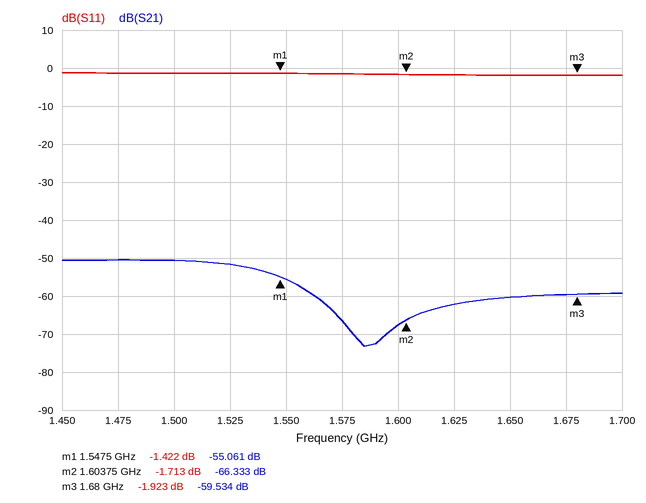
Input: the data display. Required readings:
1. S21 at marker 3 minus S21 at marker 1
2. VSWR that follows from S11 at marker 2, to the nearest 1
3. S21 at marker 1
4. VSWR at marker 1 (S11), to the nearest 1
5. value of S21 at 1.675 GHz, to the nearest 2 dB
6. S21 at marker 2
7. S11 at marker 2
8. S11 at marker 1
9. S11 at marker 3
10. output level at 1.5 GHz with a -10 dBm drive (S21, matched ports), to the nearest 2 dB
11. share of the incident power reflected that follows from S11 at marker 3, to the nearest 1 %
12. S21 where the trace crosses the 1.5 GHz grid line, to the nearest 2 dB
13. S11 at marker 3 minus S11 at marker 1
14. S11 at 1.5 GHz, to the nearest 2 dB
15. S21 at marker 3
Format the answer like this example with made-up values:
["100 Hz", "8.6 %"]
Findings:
["-4.473 dB", "10", "-55.061 dB", "12", "-60 dB", "-66.333 dB", "-1.713 dB", "-1.422 dB", "-1.923 dB", "-60 dBm", "64 %", "-50 dB", "-0.501 dB", "-2 dB", "-59.534 dB"]
